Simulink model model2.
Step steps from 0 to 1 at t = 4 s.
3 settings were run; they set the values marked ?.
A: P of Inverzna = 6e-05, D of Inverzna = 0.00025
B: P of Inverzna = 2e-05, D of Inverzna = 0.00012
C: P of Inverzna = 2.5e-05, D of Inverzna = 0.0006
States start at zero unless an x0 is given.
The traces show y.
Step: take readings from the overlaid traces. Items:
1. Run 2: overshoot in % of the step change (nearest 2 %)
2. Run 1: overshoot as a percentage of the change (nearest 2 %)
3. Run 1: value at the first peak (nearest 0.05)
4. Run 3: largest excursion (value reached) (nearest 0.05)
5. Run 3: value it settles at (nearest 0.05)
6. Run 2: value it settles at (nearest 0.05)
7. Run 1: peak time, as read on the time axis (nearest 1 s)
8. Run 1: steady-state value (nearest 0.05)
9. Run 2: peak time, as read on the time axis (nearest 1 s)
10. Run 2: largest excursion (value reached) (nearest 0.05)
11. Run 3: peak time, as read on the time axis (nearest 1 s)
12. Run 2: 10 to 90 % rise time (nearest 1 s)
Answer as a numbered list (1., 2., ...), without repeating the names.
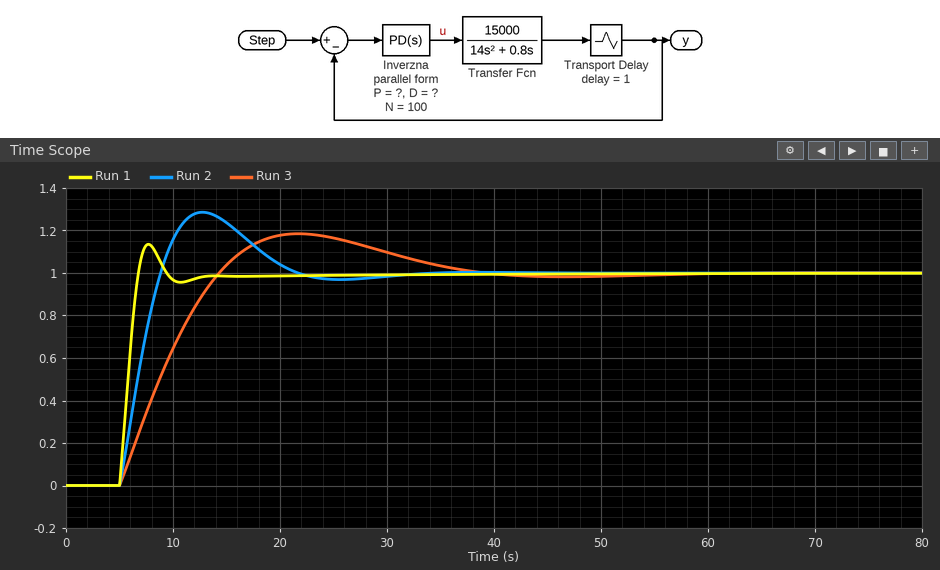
1. 28 %
2. 14 %
3. 1.15
4. 1.20
5. 1.00
6. 1.00
7. 8 s
8. 1.00
9. 13 s
10. 1.30
11. 22 s
12. 3 s
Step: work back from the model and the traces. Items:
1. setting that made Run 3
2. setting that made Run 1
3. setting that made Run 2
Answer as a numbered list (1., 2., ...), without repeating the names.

1. B
2. C
3. A
